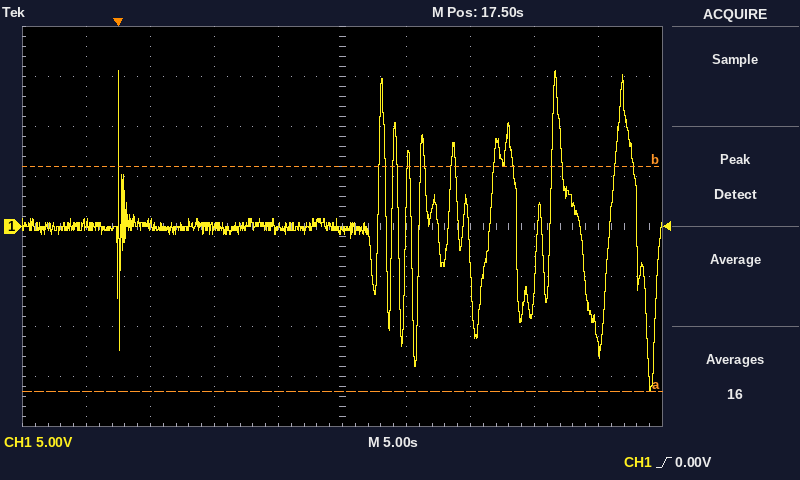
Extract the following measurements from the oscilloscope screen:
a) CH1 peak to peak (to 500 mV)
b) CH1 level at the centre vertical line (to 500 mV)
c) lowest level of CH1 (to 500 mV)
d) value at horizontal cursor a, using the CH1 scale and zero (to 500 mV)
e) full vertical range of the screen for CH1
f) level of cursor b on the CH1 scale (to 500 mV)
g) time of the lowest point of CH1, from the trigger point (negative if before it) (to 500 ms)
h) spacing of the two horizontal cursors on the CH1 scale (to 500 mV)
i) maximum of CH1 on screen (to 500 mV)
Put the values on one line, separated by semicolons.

32.0 V; -500 mV; -16.5 V; -16.5 V; 40 V; 6.0 V; +41.5 s; 22.5 V; 15.5 V
